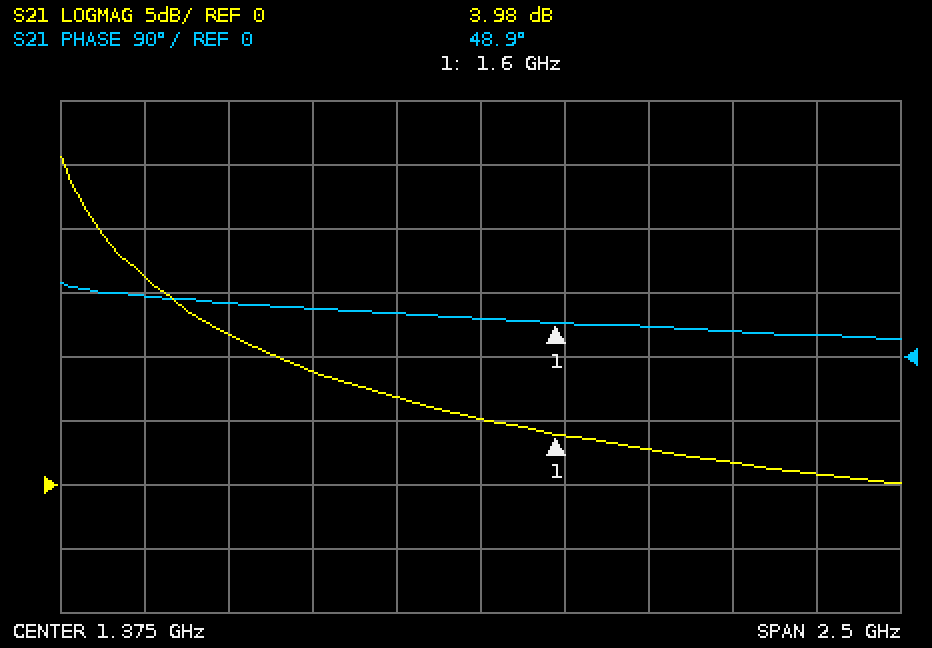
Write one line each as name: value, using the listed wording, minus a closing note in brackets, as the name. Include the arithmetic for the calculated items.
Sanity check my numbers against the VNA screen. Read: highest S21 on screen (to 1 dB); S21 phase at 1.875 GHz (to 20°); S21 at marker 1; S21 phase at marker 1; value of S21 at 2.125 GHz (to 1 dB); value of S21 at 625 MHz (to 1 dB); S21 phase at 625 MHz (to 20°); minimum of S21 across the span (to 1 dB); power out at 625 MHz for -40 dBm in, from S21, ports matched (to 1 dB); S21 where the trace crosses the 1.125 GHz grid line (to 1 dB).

highest S21 on screen: 26 dB
S21 phase at 1.875 GHz: 40°
S21 at marker 1: 3.98 dB
S21 phase at marker 1: 48.9°
value of S21 at 2.125 GHz: 2 dB
value of S21 at 625 MHz: 12 dB
S21 phase at 625 MHz: 80°
minimum of S21 across the span: 0 dB
power out at 625 MHz for -40 dBm in, from S21, ports matched: -40 dBm + (12 dB) = -28 dBm
S21 where the trace crosses the 1.125 GHz grid line: 7 dB
